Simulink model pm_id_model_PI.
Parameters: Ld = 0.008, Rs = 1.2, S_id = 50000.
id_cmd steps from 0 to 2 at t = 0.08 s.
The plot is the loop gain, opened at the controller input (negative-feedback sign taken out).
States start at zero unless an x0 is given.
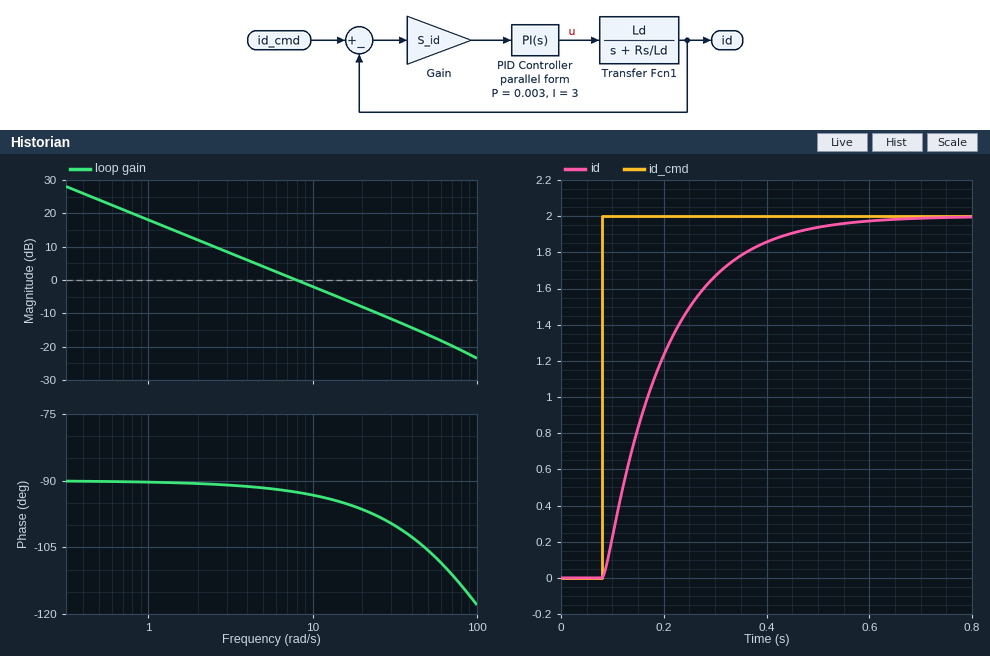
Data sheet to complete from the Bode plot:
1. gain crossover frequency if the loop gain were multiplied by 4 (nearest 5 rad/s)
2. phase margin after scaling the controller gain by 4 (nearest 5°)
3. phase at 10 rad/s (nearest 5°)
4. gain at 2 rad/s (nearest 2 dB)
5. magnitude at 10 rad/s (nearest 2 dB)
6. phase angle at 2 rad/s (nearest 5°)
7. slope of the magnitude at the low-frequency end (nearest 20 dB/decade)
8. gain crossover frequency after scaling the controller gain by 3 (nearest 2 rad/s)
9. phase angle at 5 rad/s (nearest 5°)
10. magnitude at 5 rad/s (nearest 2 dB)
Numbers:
30 rad/s
80°
-95°
12 dB
-2 dB
-90°
-20 dB/decade
24 rad/s
-90°
4 dB
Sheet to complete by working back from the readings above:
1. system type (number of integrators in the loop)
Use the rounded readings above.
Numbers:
1
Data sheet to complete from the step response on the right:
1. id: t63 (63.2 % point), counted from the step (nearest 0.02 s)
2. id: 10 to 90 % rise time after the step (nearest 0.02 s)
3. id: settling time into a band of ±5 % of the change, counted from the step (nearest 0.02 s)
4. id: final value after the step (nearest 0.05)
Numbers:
0.12 s
0.26 s
0.36 s
2.00
